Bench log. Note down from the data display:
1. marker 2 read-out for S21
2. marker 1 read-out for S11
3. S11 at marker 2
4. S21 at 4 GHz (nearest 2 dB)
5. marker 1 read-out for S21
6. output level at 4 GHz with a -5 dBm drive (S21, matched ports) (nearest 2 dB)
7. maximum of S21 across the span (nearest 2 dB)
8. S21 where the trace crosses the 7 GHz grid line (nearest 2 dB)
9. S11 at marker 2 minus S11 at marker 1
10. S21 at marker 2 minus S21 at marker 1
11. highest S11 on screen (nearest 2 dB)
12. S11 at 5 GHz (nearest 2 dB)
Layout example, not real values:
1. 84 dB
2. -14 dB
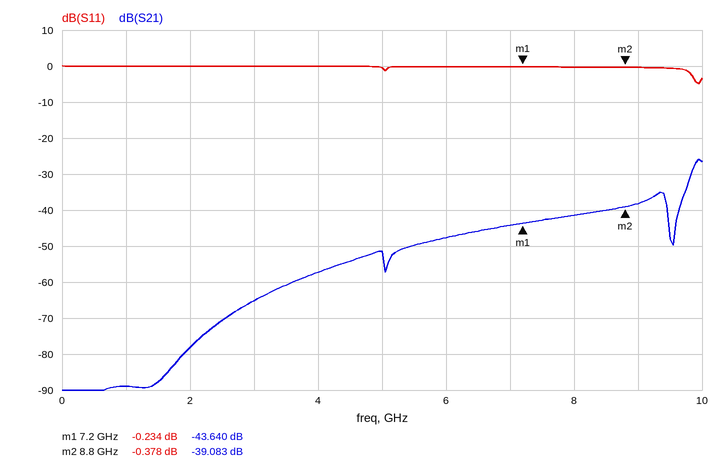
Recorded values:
1. -39.083 dB
2. -0.234 dB
3. -0.378 dB
4. -58 dB
5. -43.640 dB
6. -62 dBm
7. -26 dB
8. -44 dB
9. -0.144 dB
10. 4.557 dB
11. 0 dB
12. 0 dB
